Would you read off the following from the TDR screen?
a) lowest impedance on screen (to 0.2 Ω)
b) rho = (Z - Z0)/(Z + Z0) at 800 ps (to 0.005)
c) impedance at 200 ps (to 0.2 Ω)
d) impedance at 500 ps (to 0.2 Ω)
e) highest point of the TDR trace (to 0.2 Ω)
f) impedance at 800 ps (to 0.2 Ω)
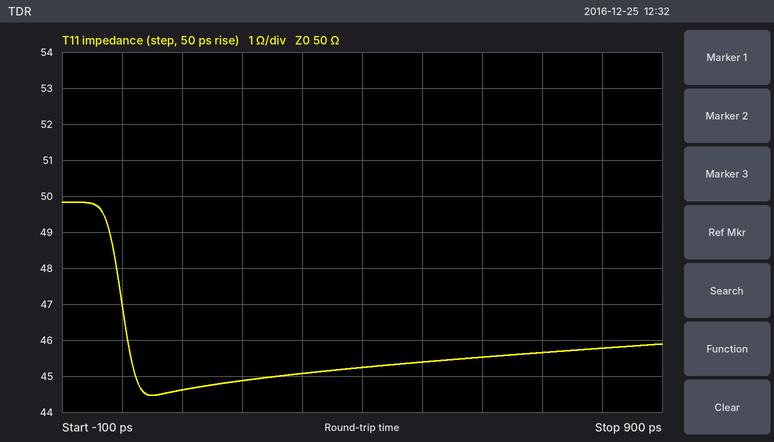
44.4 Ω
-0.045
44.8 Ω
45.4 Ω
49.8 Ω
45.8 Ω
